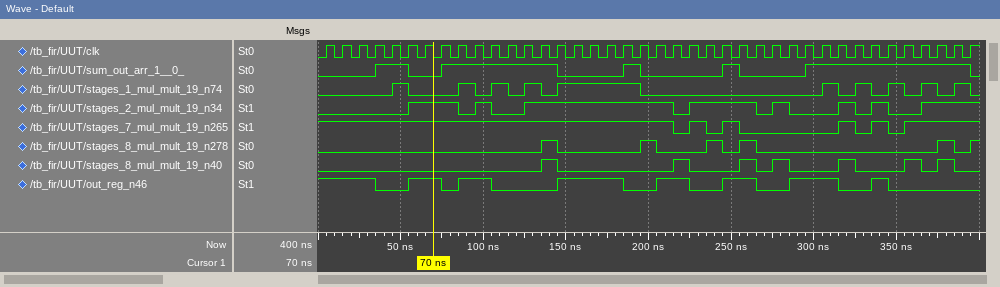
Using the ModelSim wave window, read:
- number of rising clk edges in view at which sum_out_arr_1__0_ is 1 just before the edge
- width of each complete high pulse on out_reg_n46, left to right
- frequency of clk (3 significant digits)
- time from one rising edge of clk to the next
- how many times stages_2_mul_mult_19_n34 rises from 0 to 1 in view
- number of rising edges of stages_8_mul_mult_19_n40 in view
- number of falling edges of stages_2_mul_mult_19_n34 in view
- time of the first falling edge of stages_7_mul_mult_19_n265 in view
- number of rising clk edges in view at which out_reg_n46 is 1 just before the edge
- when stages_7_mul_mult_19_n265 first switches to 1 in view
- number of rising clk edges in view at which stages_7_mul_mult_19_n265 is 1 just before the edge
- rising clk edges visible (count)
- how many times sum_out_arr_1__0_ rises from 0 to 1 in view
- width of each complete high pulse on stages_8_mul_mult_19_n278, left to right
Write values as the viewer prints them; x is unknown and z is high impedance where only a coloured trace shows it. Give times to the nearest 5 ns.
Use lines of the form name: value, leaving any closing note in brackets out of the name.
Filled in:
number of rising clk edges in view at which sum_out_arr_1__0_ is 1 just before the edge: 21
width of each complete high pulse on out_reg_n46, left to right: 20 ns, 20 ns, 40 ns, 20 ns, 20 ns, 30 ns, 10 ns
frequency of clk: 100 MHz
time from one rising edge of clk to the next: 10 ns
how many times stages_2_mul_mult_19_n34 rises from 0 to 1 in view: 8
number of rising edges of stages_8_mul_mult_19_n40 in view: 7
number of falling edges of stages_2_mul_mult_19_n34 in view: 7
time of the first falling edge of stages_7_mul_mult_19_n265 in view: 215 ns
number of rising clk edges in view at which out_reg_n46 is 1 just before the edge: 20
when stages_7_mul_mult_19_n265 first switches to 1 in view: 225 ns
number of rising clk edges in view at which stages_7_mul_mult_19_n265 is 1 just before the edge: 30
rising clk edges visible: 40
how many times sum_out_arr_1__0_ rises from 0 to 1 in view: 5
width of each complete high pulse on stages_8_mul_mult_19_n278, left to right: 10 ns, 10 ns, 10 ns, 10 ns, 10 ns
